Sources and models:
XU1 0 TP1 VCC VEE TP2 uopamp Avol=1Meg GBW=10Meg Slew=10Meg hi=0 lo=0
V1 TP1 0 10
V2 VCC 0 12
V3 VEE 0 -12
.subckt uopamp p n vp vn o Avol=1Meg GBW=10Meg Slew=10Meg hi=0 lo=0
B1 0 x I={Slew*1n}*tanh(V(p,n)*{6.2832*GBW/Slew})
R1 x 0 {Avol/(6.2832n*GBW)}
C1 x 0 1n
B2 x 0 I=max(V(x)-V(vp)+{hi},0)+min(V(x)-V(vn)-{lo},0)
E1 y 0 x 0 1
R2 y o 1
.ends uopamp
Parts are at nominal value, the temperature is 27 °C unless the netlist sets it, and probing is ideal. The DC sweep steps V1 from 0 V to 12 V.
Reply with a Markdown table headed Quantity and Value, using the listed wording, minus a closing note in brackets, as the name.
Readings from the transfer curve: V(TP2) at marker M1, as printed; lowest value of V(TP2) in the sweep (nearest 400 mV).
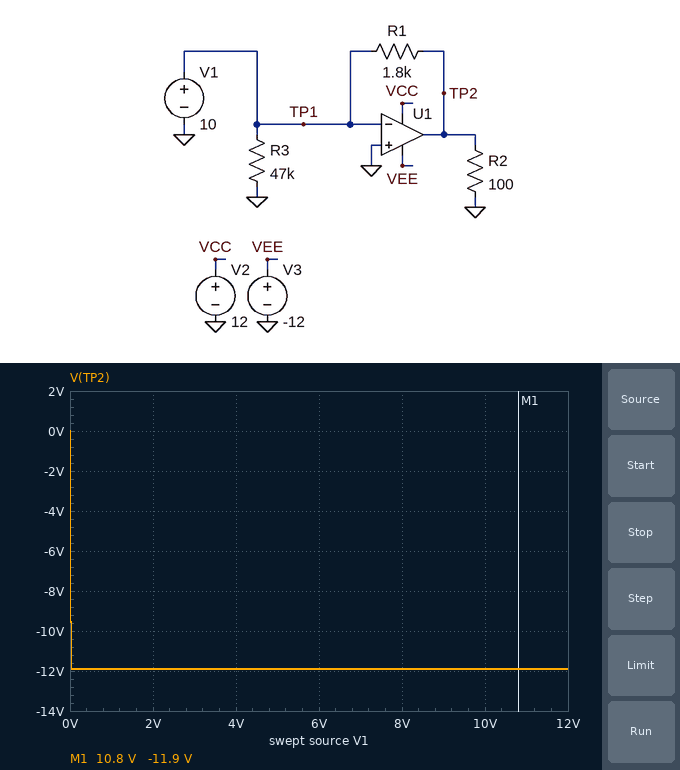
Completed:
| Quantity | Value |
|---|---|
| V(TP2) at marker M1, as printed | -11.9 V |
| lowest value of V(TP2) in the sweep | -12.0 V |
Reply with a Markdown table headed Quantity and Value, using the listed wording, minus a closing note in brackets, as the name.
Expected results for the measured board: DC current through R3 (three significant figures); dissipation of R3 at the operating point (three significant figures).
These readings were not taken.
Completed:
| Quantity | Value |
|---|---|
| DC current through R3 | 213 µA |
| dissipation of R3 at the operating point | 2.13 mW |
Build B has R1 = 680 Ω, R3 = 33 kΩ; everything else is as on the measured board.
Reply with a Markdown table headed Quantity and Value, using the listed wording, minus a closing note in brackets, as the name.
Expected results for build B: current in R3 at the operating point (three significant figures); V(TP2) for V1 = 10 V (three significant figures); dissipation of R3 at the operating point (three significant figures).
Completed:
| Quantity | Value |
|---|---|
| current in R3 at the operating point | 303 µA |
| V(TP2) for V1 = 10 V | -11.9 V |
| dissipation of R3 at the operating point | 3.03 mW |
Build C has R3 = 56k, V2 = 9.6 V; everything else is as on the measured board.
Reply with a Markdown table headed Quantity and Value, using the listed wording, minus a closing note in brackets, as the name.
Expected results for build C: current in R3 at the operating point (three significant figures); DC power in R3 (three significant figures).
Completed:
| Quantity | Value |
|---|---|
| current in R3 at the operating point | 179 µA |
| DC power in R3 | 1.79 mW |
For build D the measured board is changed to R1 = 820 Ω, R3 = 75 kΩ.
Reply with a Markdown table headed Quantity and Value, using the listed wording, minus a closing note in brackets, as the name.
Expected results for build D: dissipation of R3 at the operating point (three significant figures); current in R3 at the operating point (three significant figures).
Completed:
| Quantity | Value |
|---|---|
| dissipation of R3 at the operating point | 1.33 mW |
| current in R3 at the operating point | 133 µA |
